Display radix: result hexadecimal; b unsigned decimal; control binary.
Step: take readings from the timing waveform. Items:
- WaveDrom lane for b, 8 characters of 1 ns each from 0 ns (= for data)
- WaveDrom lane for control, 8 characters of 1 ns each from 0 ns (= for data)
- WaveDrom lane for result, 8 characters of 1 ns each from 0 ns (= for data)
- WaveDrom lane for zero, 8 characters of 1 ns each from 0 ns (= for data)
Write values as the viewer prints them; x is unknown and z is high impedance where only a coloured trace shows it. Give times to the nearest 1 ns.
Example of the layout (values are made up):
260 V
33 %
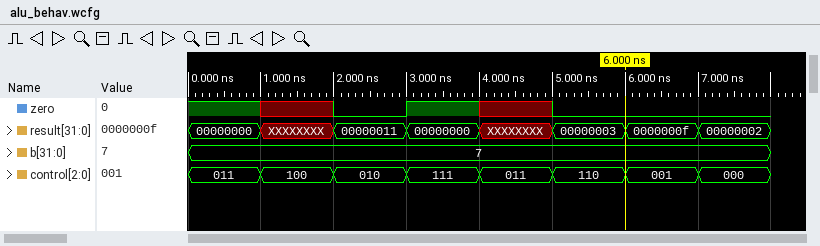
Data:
{name: 'b', wave: '=.......', data: '7'}
{name: 'control', wave: '========', data: '011 100 010 111 011 110 001 000'}
{name: 'result', wave: '=x==x===', data: '00000000 00000011 00000000 00000003 0000000f 00000002'}
{name: 'zero', wave: '1x01x0..'}
